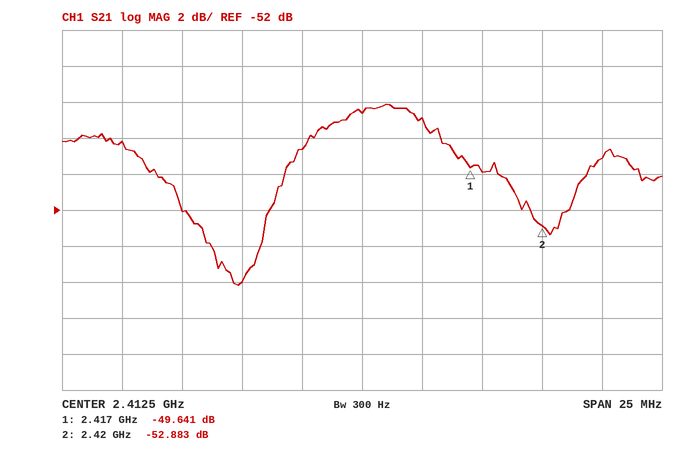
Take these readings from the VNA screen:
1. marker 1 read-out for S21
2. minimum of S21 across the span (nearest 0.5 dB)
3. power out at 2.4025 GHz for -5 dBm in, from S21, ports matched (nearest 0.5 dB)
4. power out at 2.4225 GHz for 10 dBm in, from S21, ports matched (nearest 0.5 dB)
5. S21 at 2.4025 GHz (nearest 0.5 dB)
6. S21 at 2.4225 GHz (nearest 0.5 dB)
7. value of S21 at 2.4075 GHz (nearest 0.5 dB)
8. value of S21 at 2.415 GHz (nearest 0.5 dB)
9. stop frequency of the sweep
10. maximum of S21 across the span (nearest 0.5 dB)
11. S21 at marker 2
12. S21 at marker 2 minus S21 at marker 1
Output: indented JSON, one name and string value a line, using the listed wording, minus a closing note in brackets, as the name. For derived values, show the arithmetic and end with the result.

{
  "marker 1 read-out for S21": "-49.641 dB",
  "minimum of S21 across the span": "-56.0 dB",
  "power out at 2.4025 GHz for -5 dBm in, from S21, ports matched": "-5 dBm + (-48.0 dB) = -53.0 dBm",
  "power out at 2.4225 GHz for 10 dBm in, from S21, ports matched": "10 dBm + (-49.0 dB) = -39.0 dBm",
  "S21 at 2.4025 GHz": "-48.0 dB",
  "S21 at 2.4225 GHz": "-49.0 dB",
  "value of S21 at 2.4075 GHz": "-56.0 dB",
  "value of S21 at 2.415 GHz": "-47.0 dB",
  "stop frequency of the sweep": "2.425 GHz",
  "maximum of S21 across the span": "-46.0 dB",
  "S21 at marker 2": "-52.883 dB",
  "S21 at marker 2 minus S21 at marker 1": "-52.883 − (-49.641) = -3.242 dB"
}
